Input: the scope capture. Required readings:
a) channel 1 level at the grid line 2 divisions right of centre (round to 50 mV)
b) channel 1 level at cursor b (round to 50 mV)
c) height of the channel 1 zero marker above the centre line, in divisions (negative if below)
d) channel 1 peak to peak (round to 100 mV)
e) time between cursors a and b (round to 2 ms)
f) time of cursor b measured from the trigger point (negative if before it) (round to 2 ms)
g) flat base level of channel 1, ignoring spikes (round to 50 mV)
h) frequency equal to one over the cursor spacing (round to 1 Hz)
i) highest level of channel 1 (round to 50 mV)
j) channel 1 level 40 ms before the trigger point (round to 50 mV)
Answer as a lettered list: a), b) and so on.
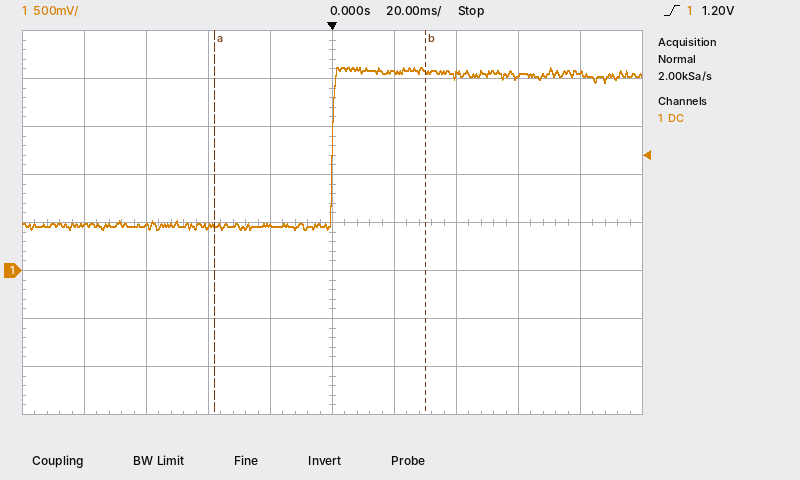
a) 2.05 V
b) 2.10 V
c) -1.0 div
d) 1.70 V
e) 68 ms
f) +30 ms
g) 450 mV
h) 15 Hz
i) 2.10 V
j) 450 mV
